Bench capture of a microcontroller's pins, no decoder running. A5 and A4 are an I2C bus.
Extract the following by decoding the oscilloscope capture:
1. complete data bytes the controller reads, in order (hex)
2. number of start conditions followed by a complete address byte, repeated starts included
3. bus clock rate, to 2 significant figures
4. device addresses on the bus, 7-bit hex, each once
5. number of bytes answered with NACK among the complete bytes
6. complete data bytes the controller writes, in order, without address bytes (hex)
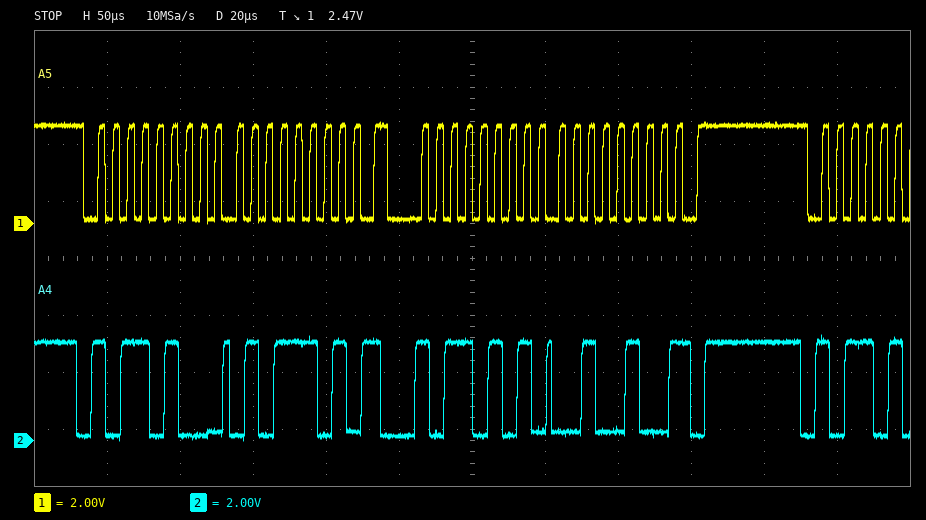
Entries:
24
2
100 kHz
0x5A
1
5D
